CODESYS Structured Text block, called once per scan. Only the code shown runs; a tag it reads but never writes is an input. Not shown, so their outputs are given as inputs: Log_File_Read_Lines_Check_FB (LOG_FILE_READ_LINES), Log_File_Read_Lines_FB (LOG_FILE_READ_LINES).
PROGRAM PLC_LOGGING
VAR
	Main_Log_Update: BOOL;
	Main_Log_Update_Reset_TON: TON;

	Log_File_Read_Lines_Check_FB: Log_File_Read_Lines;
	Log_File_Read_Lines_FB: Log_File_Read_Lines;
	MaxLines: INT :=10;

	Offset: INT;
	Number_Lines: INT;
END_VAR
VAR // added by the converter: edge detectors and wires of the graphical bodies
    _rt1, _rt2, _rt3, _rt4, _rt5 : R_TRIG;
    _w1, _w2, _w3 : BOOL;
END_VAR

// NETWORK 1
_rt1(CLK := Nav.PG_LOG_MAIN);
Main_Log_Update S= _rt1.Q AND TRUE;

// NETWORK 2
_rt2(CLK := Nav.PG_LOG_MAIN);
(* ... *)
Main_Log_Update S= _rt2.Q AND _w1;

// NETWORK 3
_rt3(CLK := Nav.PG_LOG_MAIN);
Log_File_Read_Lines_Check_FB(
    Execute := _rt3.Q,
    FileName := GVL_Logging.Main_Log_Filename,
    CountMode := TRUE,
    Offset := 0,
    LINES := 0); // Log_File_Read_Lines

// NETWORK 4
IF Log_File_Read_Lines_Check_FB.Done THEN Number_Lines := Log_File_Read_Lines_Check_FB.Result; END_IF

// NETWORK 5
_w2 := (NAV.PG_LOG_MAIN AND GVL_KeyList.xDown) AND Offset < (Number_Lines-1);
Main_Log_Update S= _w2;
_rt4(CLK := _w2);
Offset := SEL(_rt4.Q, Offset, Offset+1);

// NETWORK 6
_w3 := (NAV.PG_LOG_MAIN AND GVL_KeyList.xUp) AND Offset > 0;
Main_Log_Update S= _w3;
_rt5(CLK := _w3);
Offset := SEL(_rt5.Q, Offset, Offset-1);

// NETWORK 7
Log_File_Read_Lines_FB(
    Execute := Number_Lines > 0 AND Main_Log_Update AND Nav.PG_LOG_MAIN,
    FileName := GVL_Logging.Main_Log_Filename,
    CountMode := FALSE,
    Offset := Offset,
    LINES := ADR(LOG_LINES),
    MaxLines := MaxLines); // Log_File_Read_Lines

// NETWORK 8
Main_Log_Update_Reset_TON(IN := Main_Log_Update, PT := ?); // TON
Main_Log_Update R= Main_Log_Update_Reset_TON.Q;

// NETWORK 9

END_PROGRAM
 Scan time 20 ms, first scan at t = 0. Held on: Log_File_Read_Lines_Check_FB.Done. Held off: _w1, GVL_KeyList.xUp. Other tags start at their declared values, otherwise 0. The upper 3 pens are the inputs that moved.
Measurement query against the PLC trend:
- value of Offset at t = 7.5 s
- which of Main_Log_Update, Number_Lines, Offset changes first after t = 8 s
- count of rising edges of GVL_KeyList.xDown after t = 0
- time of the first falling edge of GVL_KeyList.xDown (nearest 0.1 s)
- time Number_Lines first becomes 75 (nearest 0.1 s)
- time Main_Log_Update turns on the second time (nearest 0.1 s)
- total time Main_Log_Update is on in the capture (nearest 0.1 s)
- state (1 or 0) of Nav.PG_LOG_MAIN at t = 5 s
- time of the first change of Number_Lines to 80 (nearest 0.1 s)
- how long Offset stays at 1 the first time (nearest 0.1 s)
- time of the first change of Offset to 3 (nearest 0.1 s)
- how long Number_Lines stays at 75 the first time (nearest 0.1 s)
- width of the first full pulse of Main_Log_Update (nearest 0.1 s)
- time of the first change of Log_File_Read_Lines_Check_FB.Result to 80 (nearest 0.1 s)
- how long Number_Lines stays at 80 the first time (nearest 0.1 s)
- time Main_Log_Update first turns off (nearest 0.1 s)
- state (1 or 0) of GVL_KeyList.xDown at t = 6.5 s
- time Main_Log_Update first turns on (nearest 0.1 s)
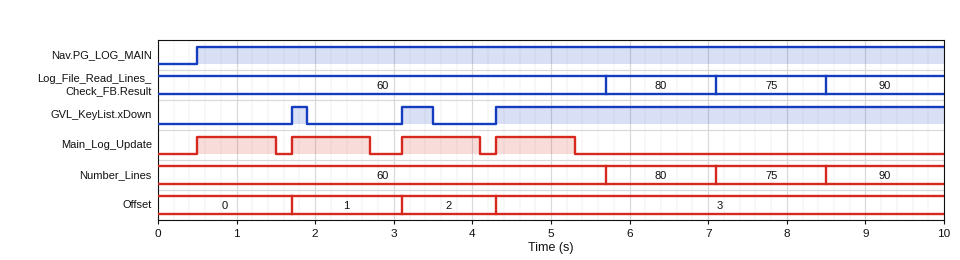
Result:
3
Number_Lines
3
1.9 s
7.1 s
1.7 s
4.0 s
1
5.7 s
1.4 s
4.3 s
1.4 s
1.0 s
5.7 s
1.4 s
1.5 s
1
0.5 s
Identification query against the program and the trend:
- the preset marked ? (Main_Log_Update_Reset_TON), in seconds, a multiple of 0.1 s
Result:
1.0 s
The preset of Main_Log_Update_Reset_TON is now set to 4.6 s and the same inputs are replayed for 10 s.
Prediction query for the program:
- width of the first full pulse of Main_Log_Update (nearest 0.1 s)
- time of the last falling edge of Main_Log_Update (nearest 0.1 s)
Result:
4.6 s
5.1 s
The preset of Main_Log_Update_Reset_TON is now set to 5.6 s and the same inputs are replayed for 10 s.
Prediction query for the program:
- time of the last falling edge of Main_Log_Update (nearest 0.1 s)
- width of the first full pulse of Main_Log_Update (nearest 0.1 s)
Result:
6.1 s
5.6 s
